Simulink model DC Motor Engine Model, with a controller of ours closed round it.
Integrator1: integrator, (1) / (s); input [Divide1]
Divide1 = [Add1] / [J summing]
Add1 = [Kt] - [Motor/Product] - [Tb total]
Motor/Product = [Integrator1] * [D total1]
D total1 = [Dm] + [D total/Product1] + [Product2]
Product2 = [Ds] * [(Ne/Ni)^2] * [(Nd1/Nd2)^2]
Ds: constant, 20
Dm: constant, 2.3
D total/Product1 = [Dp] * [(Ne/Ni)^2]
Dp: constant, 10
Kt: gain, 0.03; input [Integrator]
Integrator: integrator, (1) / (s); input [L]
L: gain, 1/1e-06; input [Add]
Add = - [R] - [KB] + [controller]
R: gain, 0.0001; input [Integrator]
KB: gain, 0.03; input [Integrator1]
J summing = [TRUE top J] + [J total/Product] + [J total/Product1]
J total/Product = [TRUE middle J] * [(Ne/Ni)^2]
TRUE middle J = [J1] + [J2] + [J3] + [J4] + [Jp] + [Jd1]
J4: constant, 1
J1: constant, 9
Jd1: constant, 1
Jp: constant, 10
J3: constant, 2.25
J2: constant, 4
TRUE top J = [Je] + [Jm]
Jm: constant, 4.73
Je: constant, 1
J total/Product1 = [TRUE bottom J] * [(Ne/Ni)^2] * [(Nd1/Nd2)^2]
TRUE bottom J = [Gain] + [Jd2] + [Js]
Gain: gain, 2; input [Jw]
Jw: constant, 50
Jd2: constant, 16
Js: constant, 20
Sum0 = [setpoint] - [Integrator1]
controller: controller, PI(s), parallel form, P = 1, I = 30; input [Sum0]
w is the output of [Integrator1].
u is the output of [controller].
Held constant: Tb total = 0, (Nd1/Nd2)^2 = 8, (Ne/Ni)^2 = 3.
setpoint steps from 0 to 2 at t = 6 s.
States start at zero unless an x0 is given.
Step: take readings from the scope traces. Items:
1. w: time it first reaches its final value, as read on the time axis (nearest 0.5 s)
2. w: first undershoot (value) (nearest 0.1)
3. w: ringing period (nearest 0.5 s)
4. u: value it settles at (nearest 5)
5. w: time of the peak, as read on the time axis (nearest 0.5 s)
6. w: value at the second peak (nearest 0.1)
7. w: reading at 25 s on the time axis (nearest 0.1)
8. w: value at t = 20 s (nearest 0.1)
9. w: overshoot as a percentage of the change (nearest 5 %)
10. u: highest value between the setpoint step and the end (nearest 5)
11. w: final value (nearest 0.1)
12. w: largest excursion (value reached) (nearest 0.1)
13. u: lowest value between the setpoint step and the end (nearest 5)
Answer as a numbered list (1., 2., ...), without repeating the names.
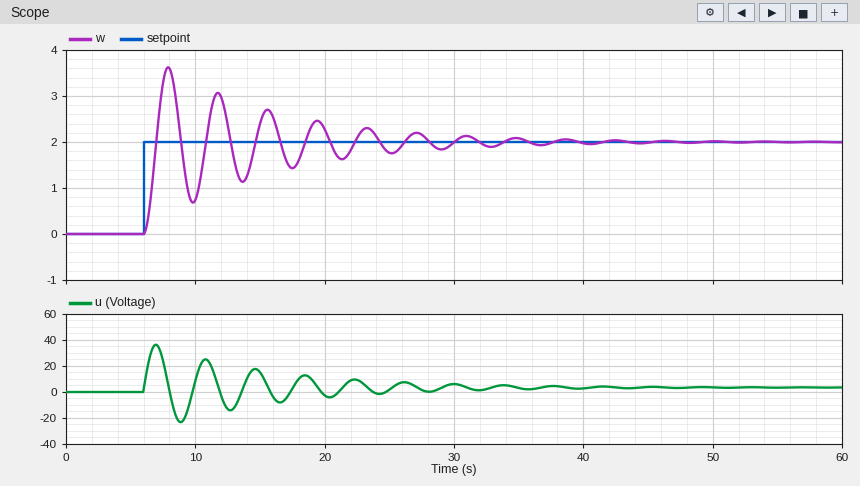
1. 7.0 s
2. 0.7
3. 4.0 s
4. 5
5. 8.0 s
6. 3.1
7. 1.8
8. 2.3
9. 80 %
10. 35
11. 2.0
12. 3.6
13. -25
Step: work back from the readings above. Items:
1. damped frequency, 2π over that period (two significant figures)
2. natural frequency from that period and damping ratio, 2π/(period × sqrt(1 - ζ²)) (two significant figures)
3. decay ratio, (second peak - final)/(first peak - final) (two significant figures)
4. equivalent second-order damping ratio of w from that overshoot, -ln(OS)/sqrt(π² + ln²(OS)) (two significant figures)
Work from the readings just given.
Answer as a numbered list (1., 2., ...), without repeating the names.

1. 1.6 rad/s
2. 1.6 rad/s
3. 0.69
4. 0.071
